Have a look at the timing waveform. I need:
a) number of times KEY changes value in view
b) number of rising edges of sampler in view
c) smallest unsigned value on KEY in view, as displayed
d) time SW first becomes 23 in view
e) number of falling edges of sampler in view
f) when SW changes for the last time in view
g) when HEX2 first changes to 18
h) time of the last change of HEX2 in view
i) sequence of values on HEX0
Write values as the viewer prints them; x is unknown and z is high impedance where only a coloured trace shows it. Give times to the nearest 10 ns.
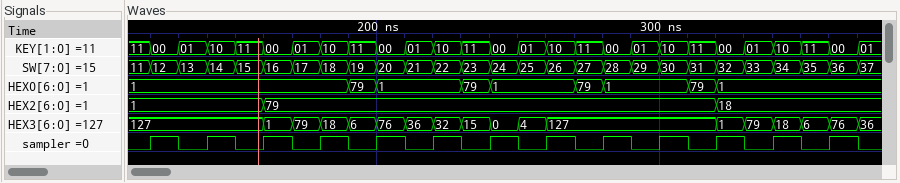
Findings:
26
13
00
230 ns
13
370 ns
320 ns
320 ns
1, 79, 1, 79, 1, 79, 1, 79, 1
